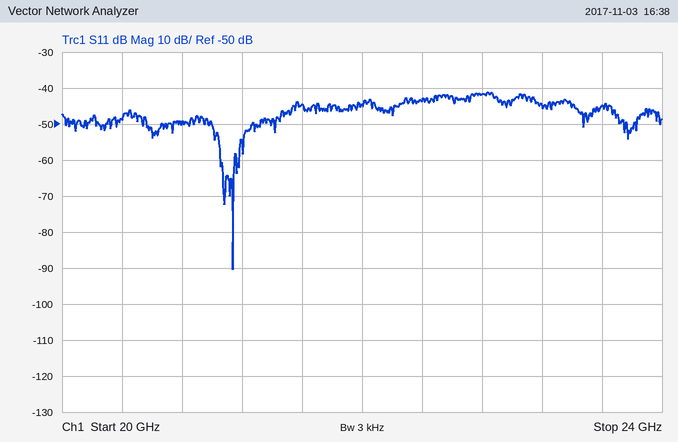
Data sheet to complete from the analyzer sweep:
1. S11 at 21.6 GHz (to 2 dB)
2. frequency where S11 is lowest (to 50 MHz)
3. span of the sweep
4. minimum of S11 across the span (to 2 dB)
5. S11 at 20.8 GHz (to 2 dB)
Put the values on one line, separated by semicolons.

-44 dB; 21.15 GHz; 4 GHz; -90 dB; -50 dB
